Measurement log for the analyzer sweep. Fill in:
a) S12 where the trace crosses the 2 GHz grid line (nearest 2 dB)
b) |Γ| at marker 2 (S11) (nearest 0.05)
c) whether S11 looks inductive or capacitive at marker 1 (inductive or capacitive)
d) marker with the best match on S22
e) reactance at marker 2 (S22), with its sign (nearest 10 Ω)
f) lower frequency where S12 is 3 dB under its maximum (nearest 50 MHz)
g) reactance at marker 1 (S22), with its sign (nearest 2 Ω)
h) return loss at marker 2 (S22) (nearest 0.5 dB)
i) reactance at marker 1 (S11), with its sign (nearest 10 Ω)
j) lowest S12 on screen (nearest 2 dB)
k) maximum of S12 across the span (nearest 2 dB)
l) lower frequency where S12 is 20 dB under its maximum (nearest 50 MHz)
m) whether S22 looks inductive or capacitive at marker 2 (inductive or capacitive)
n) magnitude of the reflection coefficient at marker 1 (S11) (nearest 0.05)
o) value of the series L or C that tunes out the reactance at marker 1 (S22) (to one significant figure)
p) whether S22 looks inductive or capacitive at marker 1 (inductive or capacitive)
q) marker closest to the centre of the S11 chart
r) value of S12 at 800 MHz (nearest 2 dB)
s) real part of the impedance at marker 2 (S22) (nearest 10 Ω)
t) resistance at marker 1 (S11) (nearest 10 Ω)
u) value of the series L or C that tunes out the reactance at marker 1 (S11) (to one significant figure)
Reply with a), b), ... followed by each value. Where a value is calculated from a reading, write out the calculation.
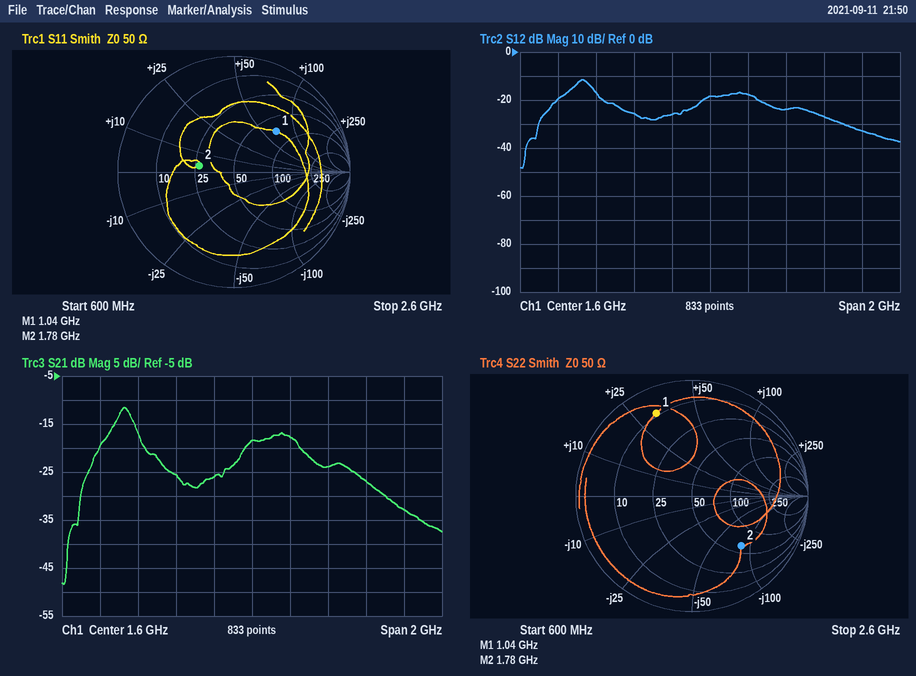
a) -24 dB
b) 0.30
c) inductive
d) marker 2
e) -80 Ω
f) 900 MHz
g) +32 Ω
h) 4.5 dB
i) +70 Ω
j) -48 dB
k) -12 dB
l) 700 MHz
m) capacitive
n) 0.50
o) C = 1/(2π × 1.04 GHz × 32 Ω) ≈ 5 pF
p) inductive
q) marker 2
r) -20 dB
s) 60 Ω
t) 70 Ω
u) C = 1/(2π × 1.04 GHz × 70 Ω) ≈ 2 pF
